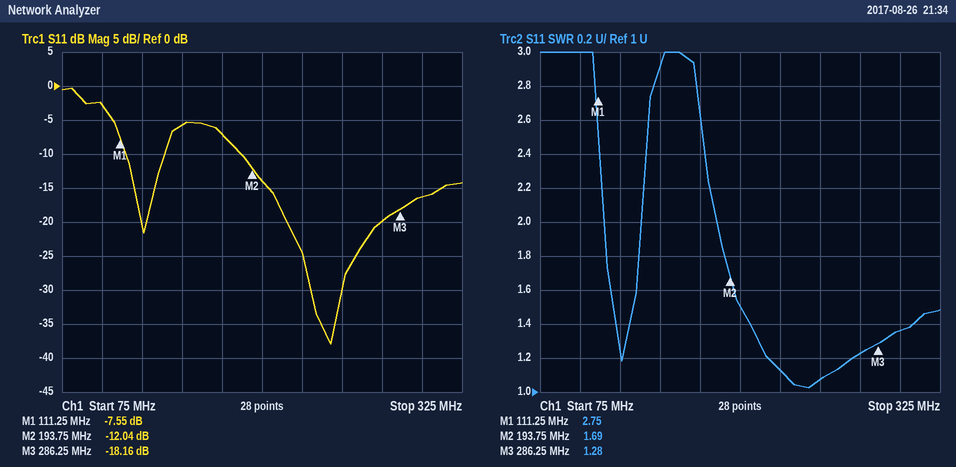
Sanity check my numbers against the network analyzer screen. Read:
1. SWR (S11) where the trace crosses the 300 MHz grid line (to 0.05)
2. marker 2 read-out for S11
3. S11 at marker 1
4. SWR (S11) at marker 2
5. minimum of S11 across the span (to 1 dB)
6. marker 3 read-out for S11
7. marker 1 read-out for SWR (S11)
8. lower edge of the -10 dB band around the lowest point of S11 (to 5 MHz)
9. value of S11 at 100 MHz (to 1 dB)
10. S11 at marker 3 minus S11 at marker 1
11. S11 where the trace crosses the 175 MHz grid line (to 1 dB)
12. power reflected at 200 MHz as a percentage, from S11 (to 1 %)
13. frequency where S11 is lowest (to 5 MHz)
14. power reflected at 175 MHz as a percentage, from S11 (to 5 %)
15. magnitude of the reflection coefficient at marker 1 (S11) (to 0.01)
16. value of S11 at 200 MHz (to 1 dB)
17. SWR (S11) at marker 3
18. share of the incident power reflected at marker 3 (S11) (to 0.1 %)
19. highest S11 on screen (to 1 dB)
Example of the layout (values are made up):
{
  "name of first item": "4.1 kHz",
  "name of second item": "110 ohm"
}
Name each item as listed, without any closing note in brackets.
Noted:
{
  "SWR (S11) where the trace crosses the 300 MHz grid line": "1.35",
  "marker 2 read-out for S11": "-12.04 dB",
  "S11 at marker 1": "-7.55 dB",
  "SWR (S11) at marker 2": "1.69",
  "minimum of S11 across the span": "-38 dB",
  "marker 3 read-out for S11": "-18.16 dB",
  "marker 1 read-out for SWR": "2.75",
  "lower edge of the -10 dB band around the lowest point of S11": "185 MHz",
  "value of S11 at 100 MHz": "-3 dB",
  "S11 at marker 3 minus S11 at marker 1": "-10.61 dB",
  "S11 where the trace crosses the 175 MHz grid line": "-7 dB",
  "power reflected at 200 MHz as a percentage, from S11": "4 %",
  "frequency where S11 is lowest": "245 MHz",
  "power reflected at 175 MHz as a percentage, from S11": "20 %",
  "magnitude of the reflection coefficient at marker 1 (S11)": "0.42",
  "value of S11 at 200 MHz": "-14 dB",
  "SWR (S11) at marker 3": "1.28",
  "share of the incident power reflected at marker 3 (S11)": "1.5 %",
  "highest S11 on screen": "0 dB"
}
